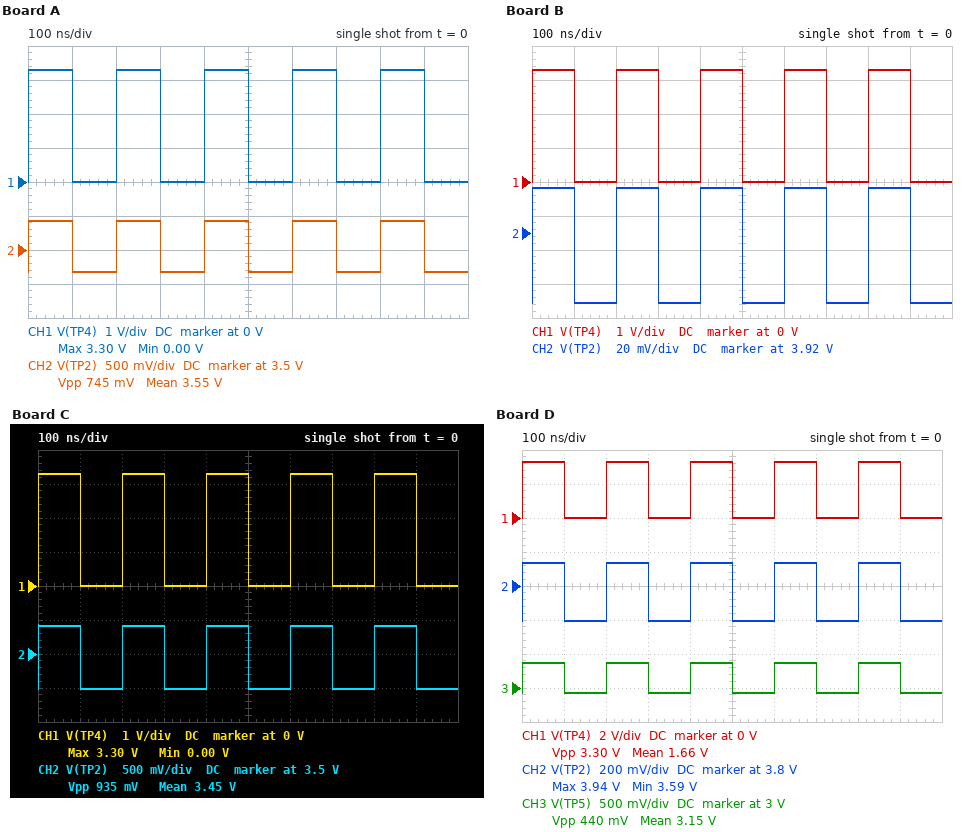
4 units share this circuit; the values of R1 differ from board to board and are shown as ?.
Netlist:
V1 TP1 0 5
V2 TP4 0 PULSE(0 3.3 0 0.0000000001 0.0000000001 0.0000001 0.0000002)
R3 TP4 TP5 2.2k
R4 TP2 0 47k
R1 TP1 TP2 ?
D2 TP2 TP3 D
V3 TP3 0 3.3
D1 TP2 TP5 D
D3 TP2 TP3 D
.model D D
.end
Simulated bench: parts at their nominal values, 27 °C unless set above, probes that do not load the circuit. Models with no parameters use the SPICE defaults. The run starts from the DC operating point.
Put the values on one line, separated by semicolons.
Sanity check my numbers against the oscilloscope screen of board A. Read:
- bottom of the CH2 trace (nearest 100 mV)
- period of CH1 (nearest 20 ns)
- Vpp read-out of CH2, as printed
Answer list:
3.2 V; 200 ns; 745 mV
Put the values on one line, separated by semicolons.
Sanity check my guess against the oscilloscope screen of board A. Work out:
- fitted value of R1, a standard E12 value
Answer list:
1.5 kΩ
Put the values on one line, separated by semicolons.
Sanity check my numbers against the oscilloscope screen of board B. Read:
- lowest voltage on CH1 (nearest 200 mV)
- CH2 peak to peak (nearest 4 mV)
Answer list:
0 V; 68 mV
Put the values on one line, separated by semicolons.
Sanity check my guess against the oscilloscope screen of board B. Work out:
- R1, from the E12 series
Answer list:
680 Ω
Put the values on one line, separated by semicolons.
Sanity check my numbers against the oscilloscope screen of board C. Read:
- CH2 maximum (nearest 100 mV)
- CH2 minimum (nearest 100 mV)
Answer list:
3.9 V; 3.0 V
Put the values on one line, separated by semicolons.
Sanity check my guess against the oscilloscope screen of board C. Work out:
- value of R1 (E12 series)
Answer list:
1.8 kΩ
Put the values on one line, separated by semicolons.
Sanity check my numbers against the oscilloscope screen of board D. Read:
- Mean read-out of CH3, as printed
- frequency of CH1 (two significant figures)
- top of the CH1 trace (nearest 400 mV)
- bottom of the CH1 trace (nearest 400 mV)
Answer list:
3.15 V; 5.0 MHz; 3.2 V; 0 V
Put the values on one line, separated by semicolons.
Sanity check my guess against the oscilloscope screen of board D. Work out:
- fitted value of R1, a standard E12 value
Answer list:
1 kΩ
